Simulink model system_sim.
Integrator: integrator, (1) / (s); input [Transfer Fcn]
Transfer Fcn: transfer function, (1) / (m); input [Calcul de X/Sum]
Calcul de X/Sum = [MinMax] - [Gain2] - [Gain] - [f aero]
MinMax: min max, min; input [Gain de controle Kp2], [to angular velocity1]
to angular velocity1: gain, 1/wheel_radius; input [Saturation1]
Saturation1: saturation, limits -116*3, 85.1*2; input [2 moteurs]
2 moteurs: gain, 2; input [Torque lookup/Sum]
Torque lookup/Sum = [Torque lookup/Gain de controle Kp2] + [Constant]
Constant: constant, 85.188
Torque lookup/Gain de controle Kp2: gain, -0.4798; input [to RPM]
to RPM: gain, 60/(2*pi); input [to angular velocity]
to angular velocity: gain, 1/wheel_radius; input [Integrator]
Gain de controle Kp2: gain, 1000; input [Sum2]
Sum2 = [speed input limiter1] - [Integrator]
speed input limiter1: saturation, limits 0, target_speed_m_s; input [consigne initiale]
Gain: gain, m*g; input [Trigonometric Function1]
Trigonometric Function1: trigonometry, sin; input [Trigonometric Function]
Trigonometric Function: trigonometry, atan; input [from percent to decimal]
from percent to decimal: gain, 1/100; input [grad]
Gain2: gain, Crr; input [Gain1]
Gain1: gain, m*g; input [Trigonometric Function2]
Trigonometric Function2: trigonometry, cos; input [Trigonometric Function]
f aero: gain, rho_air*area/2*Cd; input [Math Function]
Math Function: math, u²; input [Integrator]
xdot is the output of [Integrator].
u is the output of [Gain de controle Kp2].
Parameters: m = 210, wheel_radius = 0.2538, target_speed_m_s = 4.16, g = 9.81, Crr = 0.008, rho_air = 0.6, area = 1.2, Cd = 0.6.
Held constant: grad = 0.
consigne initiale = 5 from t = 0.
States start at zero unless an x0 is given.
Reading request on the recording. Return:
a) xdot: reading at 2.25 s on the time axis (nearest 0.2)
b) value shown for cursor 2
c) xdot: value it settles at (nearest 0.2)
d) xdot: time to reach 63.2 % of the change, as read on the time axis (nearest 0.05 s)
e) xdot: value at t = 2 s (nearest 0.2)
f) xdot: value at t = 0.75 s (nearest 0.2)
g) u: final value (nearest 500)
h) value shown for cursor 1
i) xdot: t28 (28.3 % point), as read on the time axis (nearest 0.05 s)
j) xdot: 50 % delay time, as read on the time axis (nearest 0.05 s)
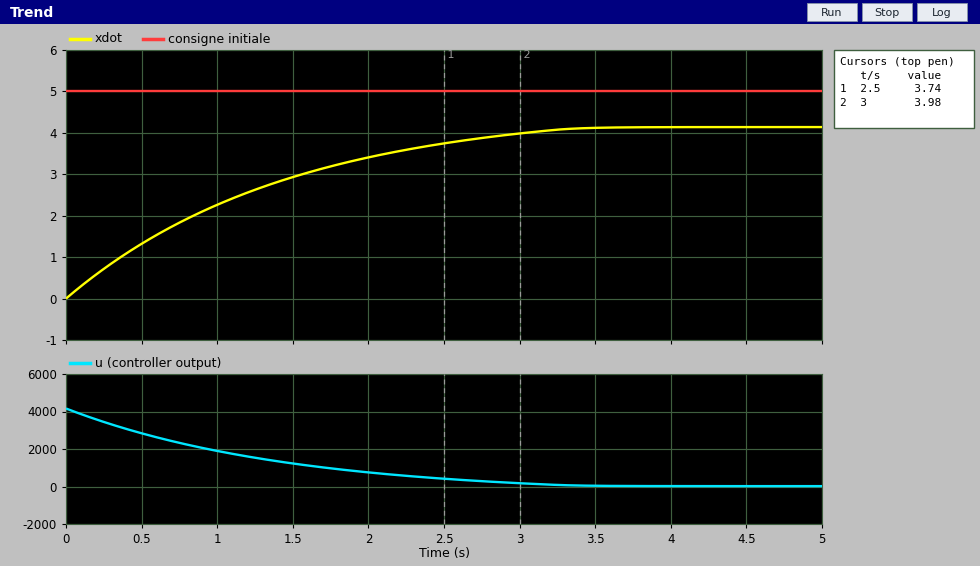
3.6
3.98
4.2
1.25 s
3.4
1.8
0
3.74
0.45 s
0.90 s
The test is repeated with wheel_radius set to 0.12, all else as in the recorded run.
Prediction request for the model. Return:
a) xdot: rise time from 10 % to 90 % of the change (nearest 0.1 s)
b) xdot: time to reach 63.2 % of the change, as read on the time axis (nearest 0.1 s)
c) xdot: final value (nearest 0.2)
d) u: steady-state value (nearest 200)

0.7 s
0.3 s
2.2
2000
